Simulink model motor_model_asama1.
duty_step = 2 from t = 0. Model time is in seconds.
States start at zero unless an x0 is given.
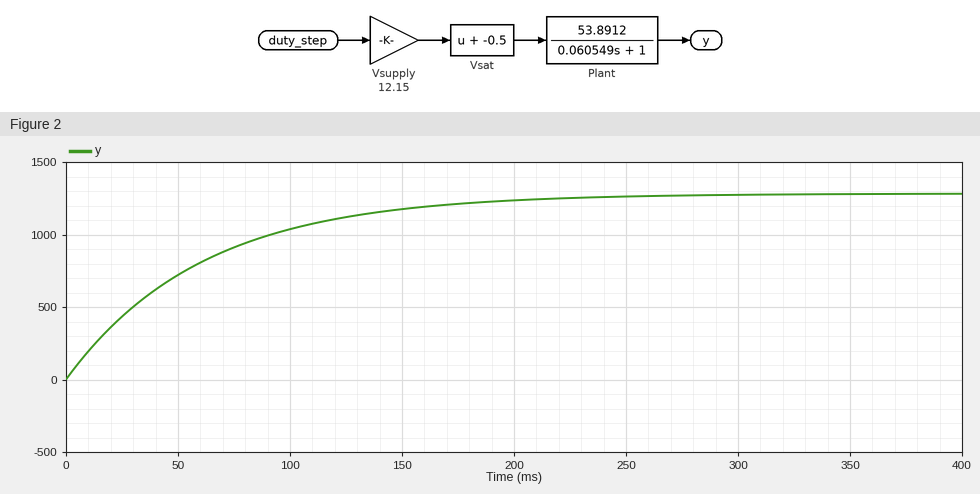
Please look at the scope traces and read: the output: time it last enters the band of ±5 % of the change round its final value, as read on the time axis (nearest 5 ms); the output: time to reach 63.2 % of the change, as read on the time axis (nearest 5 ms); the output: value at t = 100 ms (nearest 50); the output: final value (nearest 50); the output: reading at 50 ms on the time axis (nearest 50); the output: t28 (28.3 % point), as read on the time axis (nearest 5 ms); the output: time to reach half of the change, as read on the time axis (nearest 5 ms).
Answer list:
180 ms
60 ms
1050
1300
700
20 ms
40 ms
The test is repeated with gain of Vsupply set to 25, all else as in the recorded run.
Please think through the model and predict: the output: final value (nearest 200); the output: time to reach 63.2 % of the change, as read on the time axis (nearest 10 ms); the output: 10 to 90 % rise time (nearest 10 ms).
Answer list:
2600
60 ms
130 ms
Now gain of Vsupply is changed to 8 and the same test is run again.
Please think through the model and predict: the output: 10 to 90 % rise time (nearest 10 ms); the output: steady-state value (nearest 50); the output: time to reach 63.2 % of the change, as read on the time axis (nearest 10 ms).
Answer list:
130 ms
850
60 ms
